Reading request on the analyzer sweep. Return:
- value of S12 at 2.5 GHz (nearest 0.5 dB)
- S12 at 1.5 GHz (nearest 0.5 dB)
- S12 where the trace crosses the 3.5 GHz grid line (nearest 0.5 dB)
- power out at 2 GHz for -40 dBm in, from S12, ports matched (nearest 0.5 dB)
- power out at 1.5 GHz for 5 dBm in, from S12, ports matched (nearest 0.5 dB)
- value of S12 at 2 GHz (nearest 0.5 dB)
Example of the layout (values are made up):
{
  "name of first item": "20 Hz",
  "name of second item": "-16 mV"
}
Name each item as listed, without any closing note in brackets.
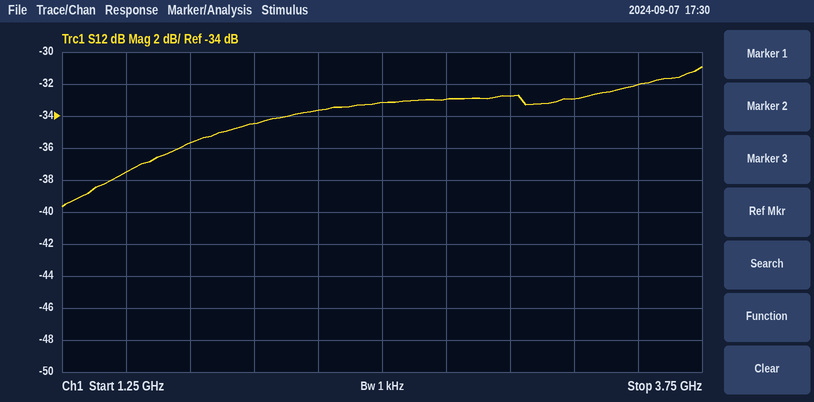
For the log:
{
  "value of S12 at 2.5 GHz": "-33.0 dB",
  "S12 at 1.5 GHz": "-37.5 dB",
  "S12 where the trace crosses the 3.5 GHz grid line": "-32.0 dB",
  "power out at 2 GHz for -40 dBm in, from S12, ports matched": "-74.5 dBm",
  "power out at 1.5 GHz for 5 dBm in, from S12, ports matched": "-32.5 dBm",
  "value of S12 at 2 GHz": "-34.5 dB"
}
